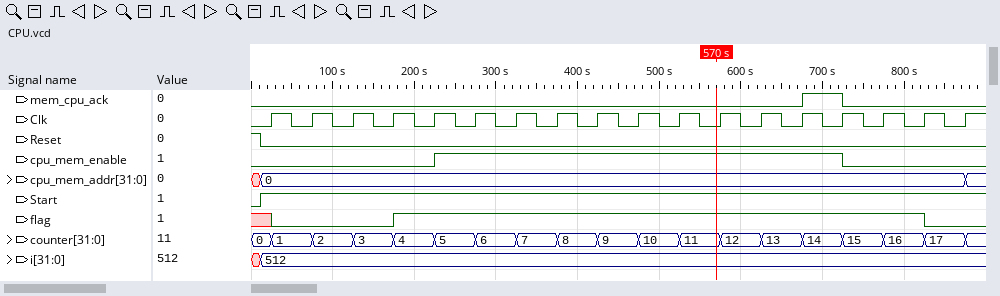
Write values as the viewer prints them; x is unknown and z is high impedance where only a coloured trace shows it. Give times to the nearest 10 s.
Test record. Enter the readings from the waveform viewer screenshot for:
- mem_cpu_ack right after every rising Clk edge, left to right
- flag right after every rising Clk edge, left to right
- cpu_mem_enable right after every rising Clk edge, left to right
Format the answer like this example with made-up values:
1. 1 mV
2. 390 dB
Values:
1. 0 0 0 0 0 0 0 0 0 0 0 0 0 1 0 0 0 0
2. 0 0 0 1 1 1 1 1 1 1 1 1 1 1 1 1 0 0
3. 0 0 0 0 1 1 1 1 1 1 1 1 1 1 0 0 0 0
